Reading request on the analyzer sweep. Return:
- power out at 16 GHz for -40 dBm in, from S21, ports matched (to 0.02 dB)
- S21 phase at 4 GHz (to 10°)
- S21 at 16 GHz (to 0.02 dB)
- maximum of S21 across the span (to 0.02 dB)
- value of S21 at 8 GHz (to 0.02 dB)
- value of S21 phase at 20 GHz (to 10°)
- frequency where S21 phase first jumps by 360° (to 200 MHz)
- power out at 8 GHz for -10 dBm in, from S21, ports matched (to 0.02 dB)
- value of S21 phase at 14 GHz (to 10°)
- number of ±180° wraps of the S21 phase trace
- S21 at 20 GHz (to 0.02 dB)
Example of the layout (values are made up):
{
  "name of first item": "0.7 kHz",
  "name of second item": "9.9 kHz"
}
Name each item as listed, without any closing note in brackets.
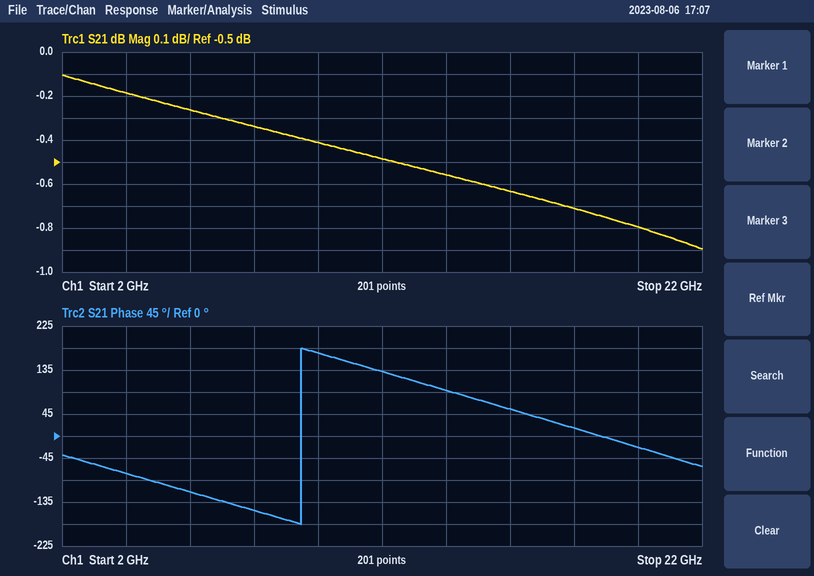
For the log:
{
  "power out at 16 GHz for -40 dBm in, from S21, ports matched": "-40.64 dBm",
  "S21 phase at 4 GHz": "-80°",
  "S21 at 16 GHz": "-0.64 dB",
  "maximum of S21 across the span": "-0.10 dB",
  "value of S21 at 8 GHz": "-0.34 dB",
  "value of S21 phase at 20 GHz": "-20°",
  "frequency where S21 phase first jumps by 360°": "9.4 GHz",
  "power out at 8 GHz for -10 dBm in, from S21, ports matched": "-10.34 dBm",
  "value of S21 phase at 14 GHz": "90°",
  "number of ±180° wraps of the S21 phase trace": "1",
  "S21 at 20 GHz": "-0.80 dB"
}
